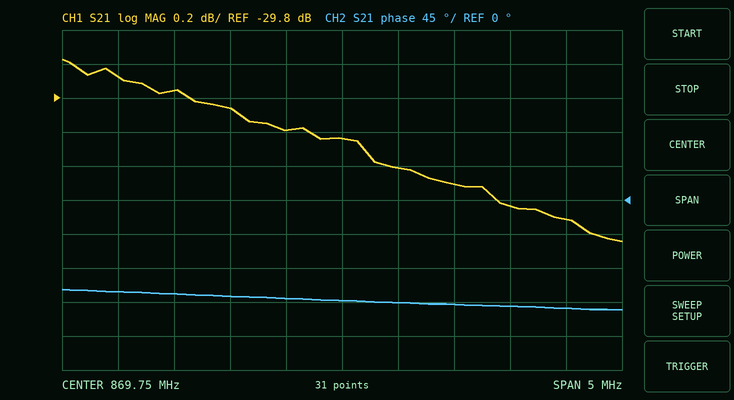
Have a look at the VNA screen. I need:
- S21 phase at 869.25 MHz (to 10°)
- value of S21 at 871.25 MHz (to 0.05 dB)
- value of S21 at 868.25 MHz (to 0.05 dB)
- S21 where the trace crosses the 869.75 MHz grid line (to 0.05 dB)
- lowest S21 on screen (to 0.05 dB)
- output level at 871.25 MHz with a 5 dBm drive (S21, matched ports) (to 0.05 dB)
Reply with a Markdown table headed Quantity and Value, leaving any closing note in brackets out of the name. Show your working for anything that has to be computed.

| Quantity | Value |
|---|---|
| S21 phase at 869.25 MHz | -130° |
| value of S21 at 871.25 MHz | -30.45 dB |
| value of S21 at 868.25 MHz | -29.75 dB |
| S21 where the trace crosses the 869.75 MHz grid line | -30.05 dB |
| lowest S21 on screen | -30.65 dB |
| output level at 871.25 MHz with a 5 dBm drive (S21, matched ports) | 5 dBm + (-30.45 dB) = -25.45 dBm |
